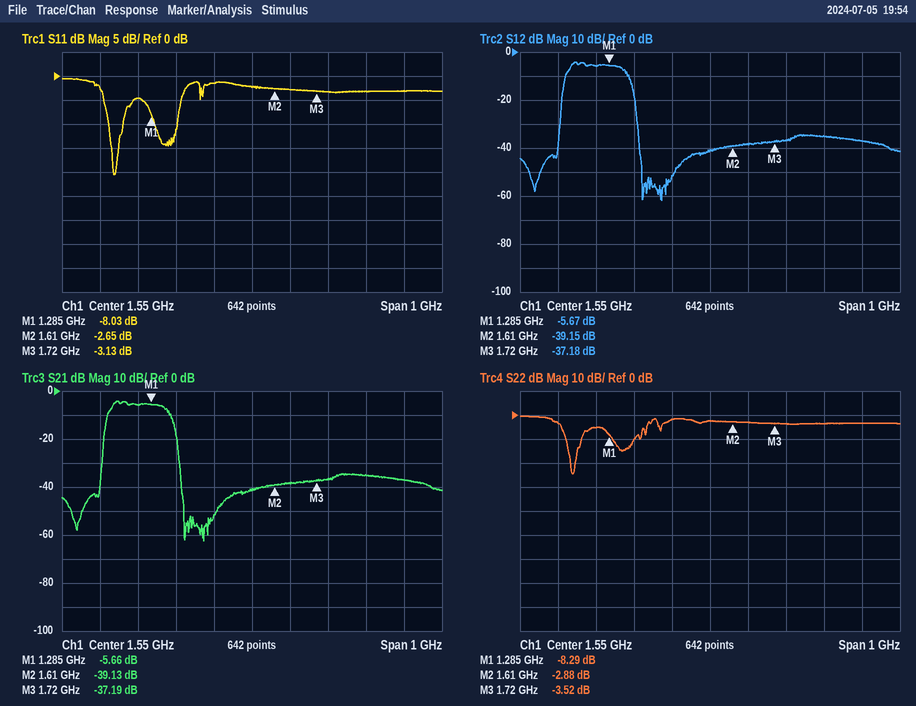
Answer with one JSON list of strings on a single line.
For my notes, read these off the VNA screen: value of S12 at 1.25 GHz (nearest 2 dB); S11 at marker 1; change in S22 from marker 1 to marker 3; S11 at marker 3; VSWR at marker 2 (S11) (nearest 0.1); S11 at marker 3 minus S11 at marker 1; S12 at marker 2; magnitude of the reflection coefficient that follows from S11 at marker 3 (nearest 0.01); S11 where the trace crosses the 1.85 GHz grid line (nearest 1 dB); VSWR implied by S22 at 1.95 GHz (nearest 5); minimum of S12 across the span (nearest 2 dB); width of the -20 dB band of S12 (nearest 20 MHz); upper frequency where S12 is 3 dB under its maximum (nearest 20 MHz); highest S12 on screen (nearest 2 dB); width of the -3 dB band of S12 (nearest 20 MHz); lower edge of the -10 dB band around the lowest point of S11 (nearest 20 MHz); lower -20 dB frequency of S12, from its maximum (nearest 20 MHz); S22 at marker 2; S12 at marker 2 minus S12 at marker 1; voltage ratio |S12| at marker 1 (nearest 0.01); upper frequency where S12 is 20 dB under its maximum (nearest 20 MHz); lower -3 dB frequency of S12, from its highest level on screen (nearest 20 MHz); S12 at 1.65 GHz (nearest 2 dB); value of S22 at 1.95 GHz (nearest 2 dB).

["-6 dB", "-8.03 dB", "4.77 dB", "-3.13 dB", "6.6", "4.90 dB", "-39.15 dB", "0.70", "-3 dB", "5", "-62 dB", "200 MHz", "1.32 GHz", "-4 dB", "140 MHz", "1.18 GHz", "1.16 GHz", "-2.88 dB", "-33.48 dB", "0.52", "1.36 GHz", "1.18 GHz", "-38 dB", "-4 dB"]
